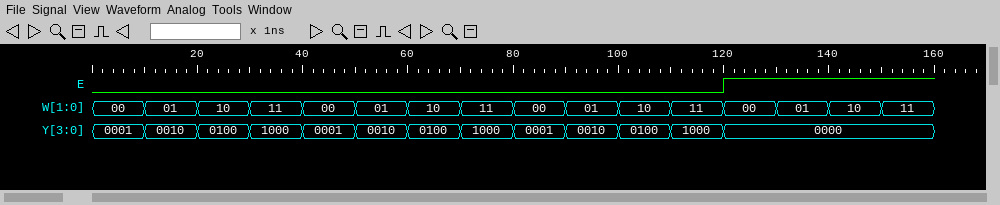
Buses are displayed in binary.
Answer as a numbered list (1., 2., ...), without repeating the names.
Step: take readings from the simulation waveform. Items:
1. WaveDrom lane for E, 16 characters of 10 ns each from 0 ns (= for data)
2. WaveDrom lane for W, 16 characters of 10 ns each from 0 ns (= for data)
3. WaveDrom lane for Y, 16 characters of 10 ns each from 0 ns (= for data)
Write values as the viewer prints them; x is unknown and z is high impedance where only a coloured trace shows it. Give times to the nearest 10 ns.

1. {name: 'E', wave: '0...........1...'}
2. {name: 'W', wave: '================', data: '00 01 10 11 00 01 10 11 00 01 10 11 00 01 10 11'}
3. {name: 'Y', wave: '=============...', data: '0001 0010 0100 1000 0001 0010 0100 1000 0001 0010 0100 1000 0000'}
